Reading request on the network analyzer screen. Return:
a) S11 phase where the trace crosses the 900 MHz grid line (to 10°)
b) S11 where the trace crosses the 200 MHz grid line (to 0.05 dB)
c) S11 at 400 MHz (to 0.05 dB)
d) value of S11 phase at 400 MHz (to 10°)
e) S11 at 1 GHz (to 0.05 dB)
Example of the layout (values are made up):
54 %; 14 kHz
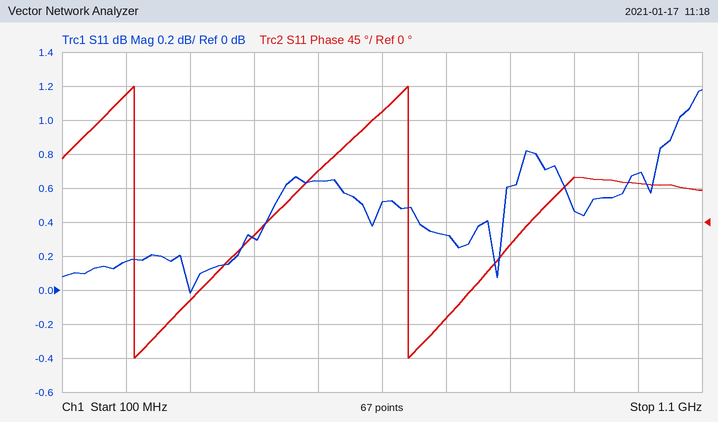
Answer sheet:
60°; 0.15 dB; 0.30 dB; -20°; 0.70 dB
